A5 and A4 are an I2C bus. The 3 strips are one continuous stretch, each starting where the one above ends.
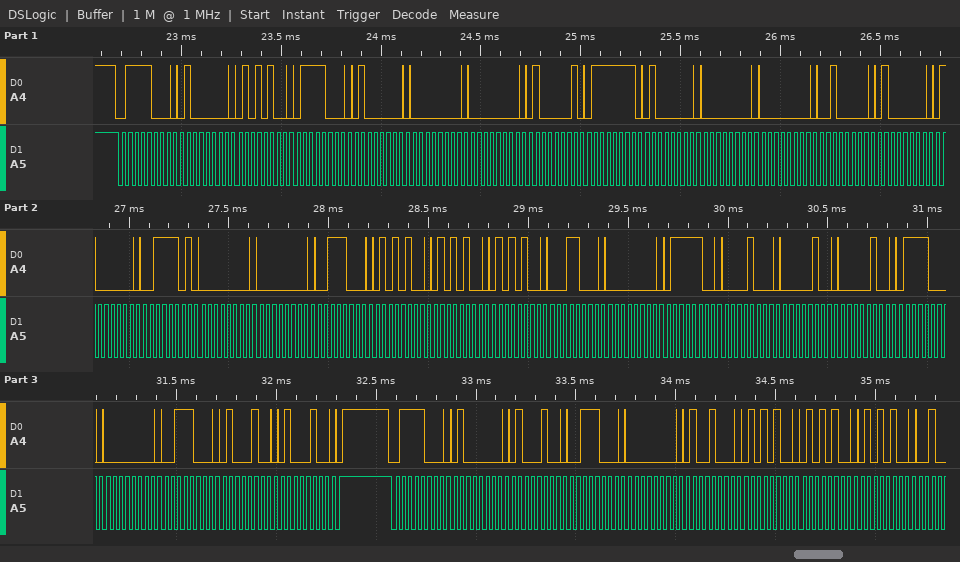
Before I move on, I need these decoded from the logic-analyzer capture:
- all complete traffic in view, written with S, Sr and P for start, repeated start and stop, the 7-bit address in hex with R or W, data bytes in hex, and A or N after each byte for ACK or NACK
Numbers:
S 3CW A 40 A 54 A 78 A 40 A 00 A 00 A 41 A 7F A 40 A 00 A 00 A 20 A 40 A 40 A 3D A 00 A 00 A 38 A 54 A 54 A 54 A 18 A 00 A 7C A 08 A 04 A 04 A 78 A 00 A 38 A 44 A 44 A P S 3CW A 40 A 44 A 38 A 00 A 48 A 54 A 54 A 54 A
